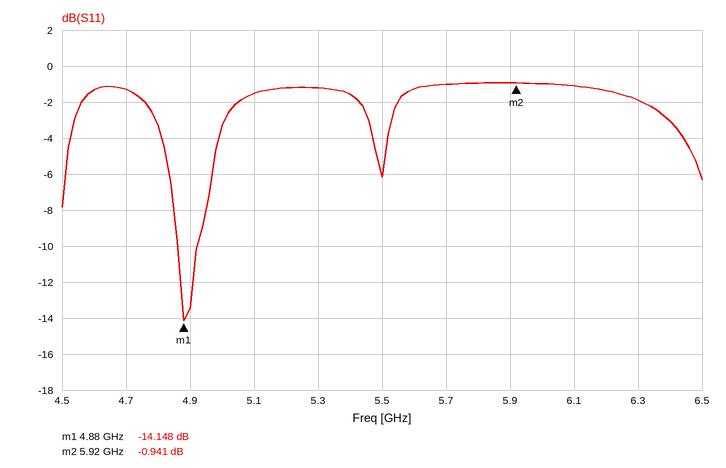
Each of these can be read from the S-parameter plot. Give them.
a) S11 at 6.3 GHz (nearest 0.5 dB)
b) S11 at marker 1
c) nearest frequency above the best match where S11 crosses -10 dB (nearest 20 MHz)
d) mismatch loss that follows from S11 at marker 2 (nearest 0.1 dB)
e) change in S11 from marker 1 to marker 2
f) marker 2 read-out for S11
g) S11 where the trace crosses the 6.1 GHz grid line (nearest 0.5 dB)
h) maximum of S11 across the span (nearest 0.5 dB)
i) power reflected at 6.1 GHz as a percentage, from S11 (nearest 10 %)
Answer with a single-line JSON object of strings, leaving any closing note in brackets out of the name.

{"S11 at 6.3 GHz": "-2.0 dB", "S11 at marker 1": "-14.148 dB", "nearest frequency above the best match where S11 crosses -10 dB": "4.92 GHz", "mismatch loss that follows from S11 at marker 2": "7.1 dB", "change in S11 from marker 1 to marker 2": "13.207 dB", "marker 2 read-out for S11": "-0.941 dB", "S11 where the trace crosses the 6.1 GHz grid line": "-1.0 dB", "maximum of S11 across the span": "-1.0 dB", "power reflected at 6.1 GHz as a percentage, from S11": "80 %"}
